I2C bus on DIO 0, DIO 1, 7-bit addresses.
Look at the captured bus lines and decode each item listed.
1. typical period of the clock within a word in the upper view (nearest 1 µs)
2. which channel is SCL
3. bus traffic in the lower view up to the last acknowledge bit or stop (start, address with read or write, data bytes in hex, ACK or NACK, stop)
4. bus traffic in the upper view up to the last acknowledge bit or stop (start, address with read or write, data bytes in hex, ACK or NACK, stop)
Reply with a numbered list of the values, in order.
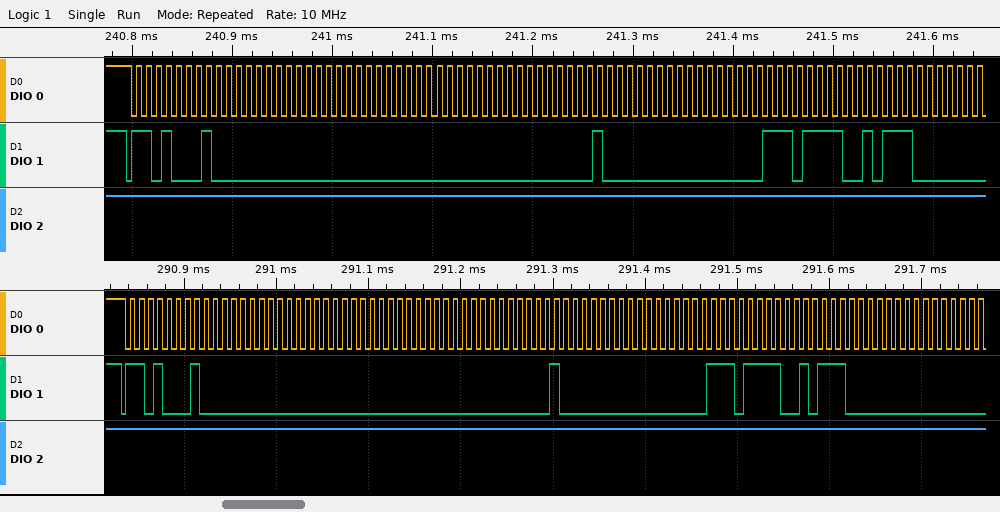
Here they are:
1. 10 µs
2. DIO 0
3. start, address 68 read ACK, 00 ACK, 00 ACK, 00 ACK, 00 ACK, 40 ACK, 00 ACK, EF ACK, 5C ACK, 00 ACK
4. start, address 68 read ACK, 00 ACK, 00 ACK, 00 ACK, 00 ACK, 40 ACK, 00 ACK, EF ACK, 5C ACK
